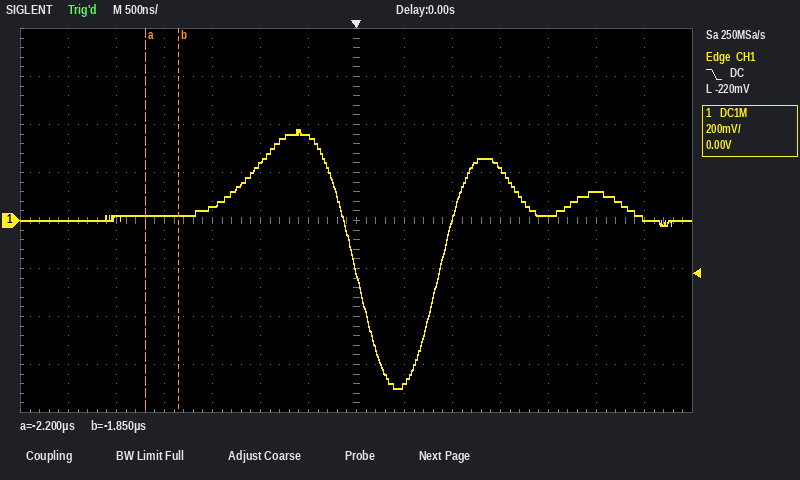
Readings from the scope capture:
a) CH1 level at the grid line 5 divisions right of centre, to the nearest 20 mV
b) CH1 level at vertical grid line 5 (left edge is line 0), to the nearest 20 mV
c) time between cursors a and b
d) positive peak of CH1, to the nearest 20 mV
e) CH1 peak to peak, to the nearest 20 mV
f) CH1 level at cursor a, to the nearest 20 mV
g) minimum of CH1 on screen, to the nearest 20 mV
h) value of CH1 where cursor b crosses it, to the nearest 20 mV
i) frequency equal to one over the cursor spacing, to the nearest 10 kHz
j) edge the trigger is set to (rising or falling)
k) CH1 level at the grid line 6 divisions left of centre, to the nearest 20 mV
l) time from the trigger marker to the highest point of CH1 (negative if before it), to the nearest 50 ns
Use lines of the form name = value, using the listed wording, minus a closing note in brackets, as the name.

CH1 level at the grid line 5 divisions right of centre, to the nearest 20 mV = 120 mV
CH1 level at vertical grid line 5 (left edge is line 0), to the nearest 20 mV = 240 mV
time between cursors a and b = 350 ns
positive peak of CH1, to the nearest 20 mV = 380 mV
CH1 peak to peak, to the nearest 20 mV = 1.08 V
CH1 level at cursor a, to the nearest 20 mV = 20 mV
minimum of CH1 on screen, to the nearest 20 mV = -700 mV
value of CH1 where cursor b crosses it, to the nearest 20 mV = 20 mV
frequency equal to one over the cursor spacing, to the nearest 10 kHz = 2.86 MHz
edge the trigger is set to = falling
CH1 level at the grid line 6 divisions left of centre, to the nearest 20 mV = 0 mV
time from the trigger marker to the highest point of CH1 (negative if before it), to the nearest 50 ns = -600 ns
